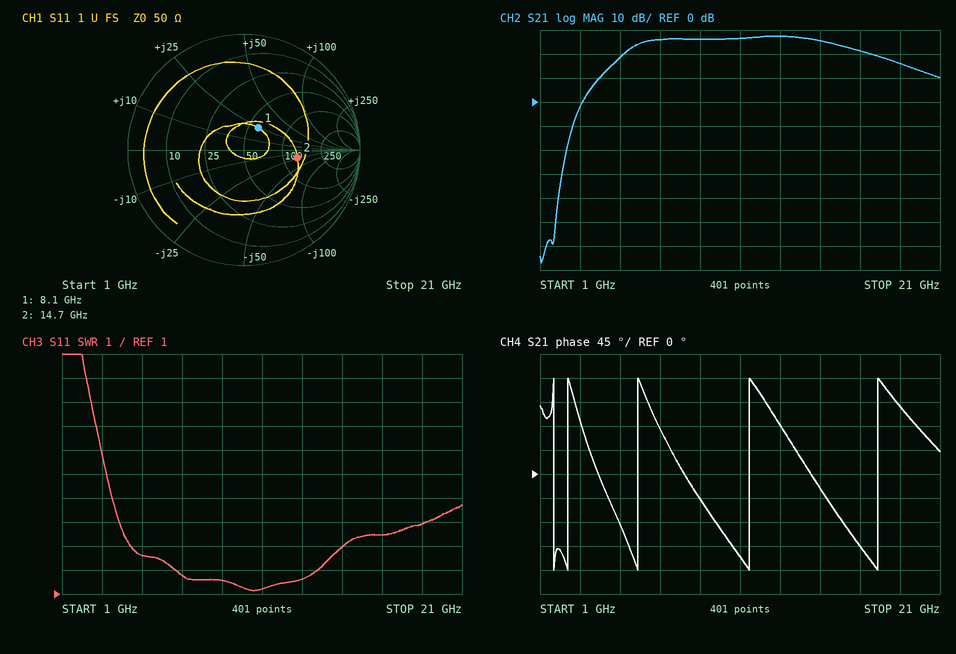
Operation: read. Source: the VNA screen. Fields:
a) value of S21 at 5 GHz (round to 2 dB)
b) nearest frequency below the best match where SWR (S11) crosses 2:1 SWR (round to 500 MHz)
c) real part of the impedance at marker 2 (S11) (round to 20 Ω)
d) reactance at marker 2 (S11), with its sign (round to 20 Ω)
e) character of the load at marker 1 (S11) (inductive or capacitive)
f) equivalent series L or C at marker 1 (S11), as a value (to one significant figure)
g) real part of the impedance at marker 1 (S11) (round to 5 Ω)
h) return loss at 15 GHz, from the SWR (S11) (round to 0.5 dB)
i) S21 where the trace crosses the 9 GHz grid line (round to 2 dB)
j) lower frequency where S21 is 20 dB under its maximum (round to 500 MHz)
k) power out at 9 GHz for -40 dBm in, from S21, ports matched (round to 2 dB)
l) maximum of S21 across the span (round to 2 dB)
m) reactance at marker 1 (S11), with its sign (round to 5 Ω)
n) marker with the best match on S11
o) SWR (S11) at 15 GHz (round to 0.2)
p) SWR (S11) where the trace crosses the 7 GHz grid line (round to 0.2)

18 dB
6.5 GHz
140 Ω
-20 Ω
inductive
500 pH
60 Ω
6.0 dB
26 dB
3.5 GHz
-14 dBm
28 dB
+25 Ω
marker 1
3.0
1.8
